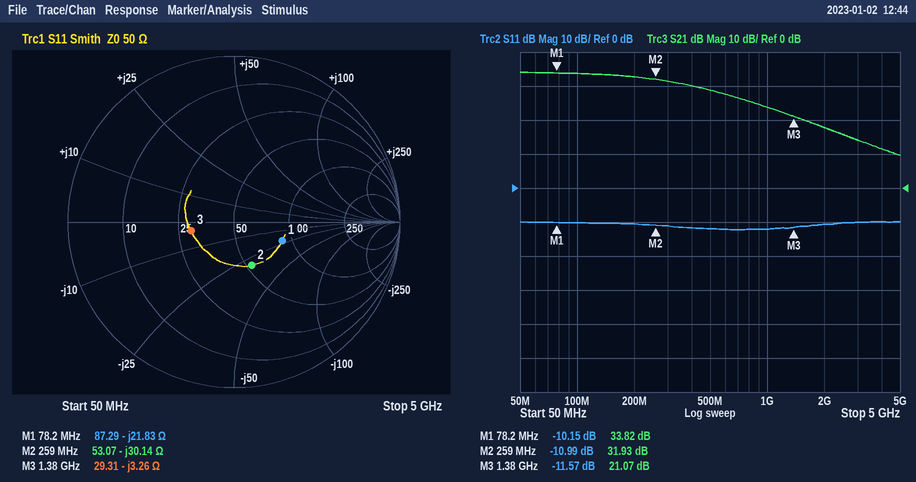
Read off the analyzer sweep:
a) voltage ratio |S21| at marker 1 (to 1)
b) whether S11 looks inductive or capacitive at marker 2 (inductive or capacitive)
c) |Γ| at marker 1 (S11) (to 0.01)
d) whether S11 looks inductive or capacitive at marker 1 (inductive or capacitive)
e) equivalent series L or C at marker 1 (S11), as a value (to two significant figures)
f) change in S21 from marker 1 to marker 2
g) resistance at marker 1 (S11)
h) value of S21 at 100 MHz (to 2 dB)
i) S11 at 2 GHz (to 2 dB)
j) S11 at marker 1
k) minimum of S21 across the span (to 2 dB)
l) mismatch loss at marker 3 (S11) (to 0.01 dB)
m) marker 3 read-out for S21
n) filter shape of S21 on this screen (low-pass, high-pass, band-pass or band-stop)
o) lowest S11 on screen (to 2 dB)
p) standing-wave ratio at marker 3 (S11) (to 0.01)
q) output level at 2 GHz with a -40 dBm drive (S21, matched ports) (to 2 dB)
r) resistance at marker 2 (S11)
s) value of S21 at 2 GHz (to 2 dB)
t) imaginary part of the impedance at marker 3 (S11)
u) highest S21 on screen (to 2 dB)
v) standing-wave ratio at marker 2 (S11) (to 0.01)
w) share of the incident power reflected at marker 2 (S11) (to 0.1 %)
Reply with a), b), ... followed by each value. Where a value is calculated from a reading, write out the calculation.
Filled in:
a) 10^(33.82/20) ≈ 49
b) capacitive
c) 0.31
d) capacitive
e) C = 1/(2π × 78.2 MHz × 21.83 Ω) ≈ 93 pF
f) 31.93 − (33.82) = -1.89 dB
g) 87.29 Ω
h) 34 dB
i) -10 dB
j) -10.15 dB
k) 10 dB
l) −10 log10(1 − 10^(-11.57/10)) ≈ 0.31 dB
m) 21.07 dB
n) low-pass
o) -12 dB
p) 1.72
q) -40 dBm + (18 dB) = -22 dBm
r) 53.07 Ω
s) 18 dB
t) -3.26 Ω
u) 34 dB
v) 1.79
w) 10^(-10.99/10) ≈ 8.0 %
